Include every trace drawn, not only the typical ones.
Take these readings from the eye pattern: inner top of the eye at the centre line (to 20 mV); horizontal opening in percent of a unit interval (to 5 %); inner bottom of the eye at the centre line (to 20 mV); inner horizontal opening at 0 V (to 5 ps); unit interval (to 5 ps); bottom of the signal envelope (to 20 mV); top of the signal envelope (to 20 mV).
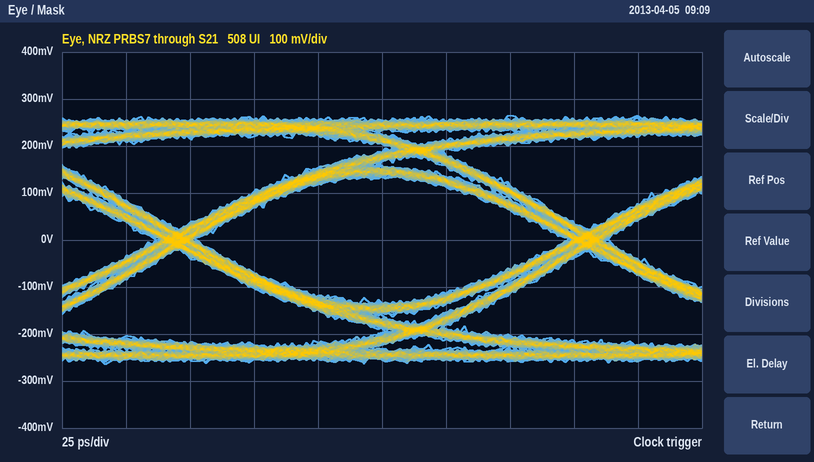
140 mV
90 %
-140 mV
145 ps
160 ps
-260 mV
260 mV
